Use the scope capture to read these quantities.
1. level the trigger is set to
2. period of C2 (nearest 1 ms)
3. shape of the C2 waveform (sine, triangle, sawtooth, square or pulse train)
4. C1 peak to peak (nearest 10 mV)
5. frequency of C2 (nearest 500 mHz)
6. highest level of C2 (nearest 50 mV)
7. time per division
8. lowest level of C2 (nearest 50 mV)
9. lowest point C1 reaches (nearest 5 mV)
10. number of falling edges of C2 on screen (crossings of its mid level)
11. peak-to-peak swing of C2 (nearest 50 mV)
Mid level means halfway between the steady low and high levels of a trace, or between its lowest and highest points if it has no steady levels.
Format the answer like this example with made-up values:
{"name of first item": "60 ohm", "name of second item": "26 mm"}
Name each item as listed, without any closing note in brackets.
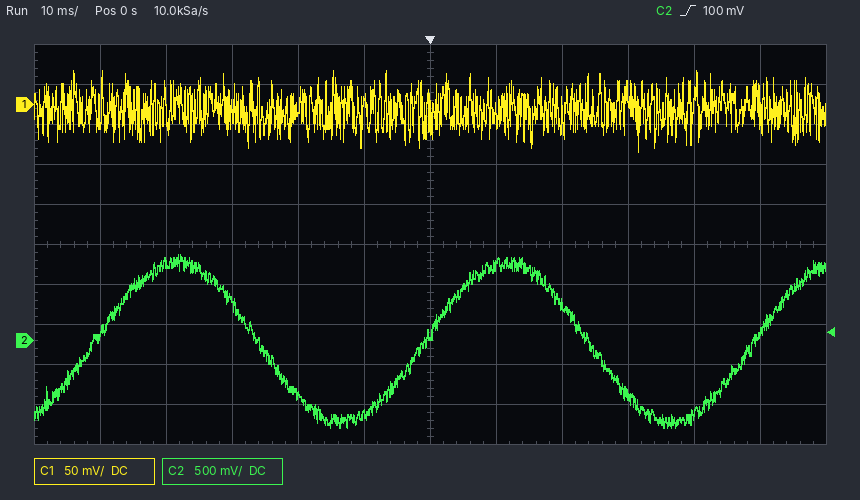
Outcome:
{"level the trigger is set to": "100 mV", "period of C2": "50 ms", "shape of the C2 waveform": "sine", "C1 peak to peak": "100 mV", "frequency of C2": "20.0 Hz", "highest level of C2": "1.05 V", "time per division": "10 ms", "lowest level of C2": "-1.10 V", "lowest point C1 reaches": "-60 mV", "number of falling edges of C2 on screen": "2", "peak-to-peak swing of C2": "2.15 V"}
